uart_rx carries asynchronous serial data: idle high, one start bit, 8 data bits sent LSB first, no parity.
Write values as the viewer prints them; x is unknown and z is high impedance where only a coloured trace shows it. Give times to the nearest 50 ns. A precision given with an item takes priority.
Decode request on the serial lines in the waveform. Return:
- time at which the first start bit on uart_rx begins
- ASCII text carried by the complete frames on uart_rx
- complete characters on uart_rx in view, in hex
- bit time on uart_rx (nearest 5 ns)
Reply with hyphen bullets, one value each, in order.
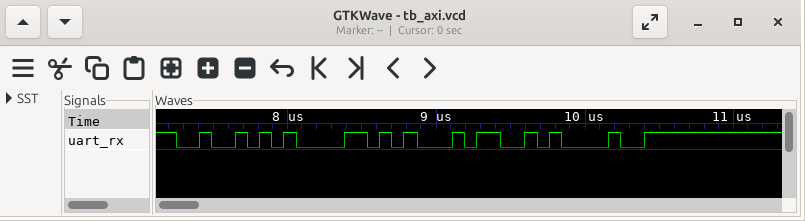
- 7250 ns
- "RX4!"
- 52, 58, 34, 21
- 80 ns
